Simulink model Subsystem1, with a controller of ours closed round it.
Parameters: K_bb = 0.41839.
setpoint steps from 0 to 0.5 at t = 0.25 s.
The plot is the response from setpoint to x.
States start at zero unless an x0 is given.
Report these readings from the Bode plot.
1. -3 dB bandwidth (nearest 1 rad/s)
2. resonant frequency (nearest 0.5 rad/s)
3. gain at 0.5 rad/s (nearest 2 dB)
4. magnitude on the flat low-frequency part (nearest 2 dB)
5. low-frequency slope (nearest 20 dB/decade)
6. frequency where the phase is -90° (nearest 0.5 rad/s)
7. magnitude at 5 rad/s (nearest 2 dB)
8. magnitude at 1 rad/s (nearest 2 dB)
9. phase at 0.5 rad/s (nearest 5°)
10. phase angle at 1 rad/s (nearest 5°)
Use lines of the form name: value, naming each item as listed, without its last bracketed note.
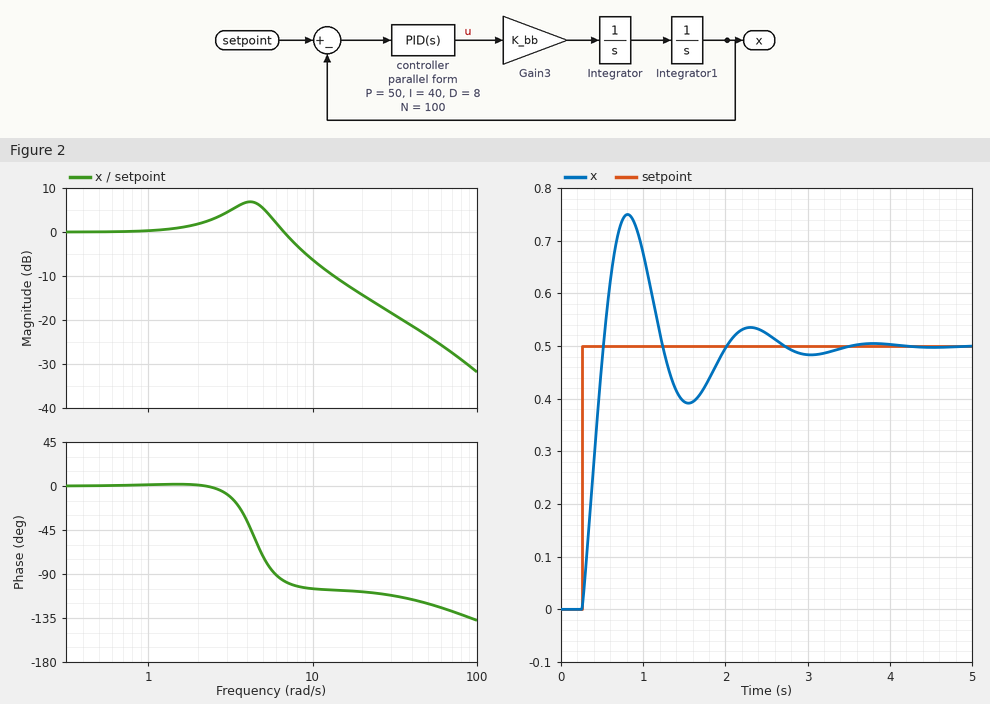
-3 dB bandwidth: 8 rad/s
resonant frequency: 4.0 rad/s
gain at 0.5 rad/s: 0 dB
magnitude on the flat low-frequency part: 0 dB
low-frequency slope: 0 dB/decade
frequency where the phase is -90°: 6.0 rad/s
magnitude at 5 rad/s: 6 dB
magnitude at 1 rad/s: 0 dB
phase at 0.5 rad/s: 0°
phase angle at 1 rad/s: 0°
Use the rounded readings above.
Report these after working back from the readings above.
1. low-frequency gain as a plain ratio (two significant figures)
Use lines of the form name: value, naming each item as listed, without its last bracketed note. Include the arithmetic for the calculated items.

low-frequency gain as a plain ratio: 10^(0 / 20) = 1.0
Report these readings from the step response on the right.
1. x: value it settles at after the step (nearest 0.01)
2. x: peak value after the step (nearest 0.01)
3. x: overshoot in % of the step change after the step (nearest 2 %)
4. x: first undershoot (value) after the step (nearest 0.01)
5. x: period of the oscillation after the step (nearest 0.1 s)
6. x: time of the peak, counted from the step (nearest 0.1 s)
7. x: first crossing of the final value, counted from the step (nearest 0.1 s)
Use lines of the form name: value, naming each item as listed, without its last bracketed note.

x: value it settles at after the step: 0.50
x: peak value after the step: 0.75
x: overshoot in % of the step change after the step: 50 %
x: first undershoot (value) after the step: 0.39
x: period of the oscillation after the step: 1.5 s
x: time of the peak, counted from the step: 0.6 s
x: first crossing of the final value, counted from the step: 0.3 s
